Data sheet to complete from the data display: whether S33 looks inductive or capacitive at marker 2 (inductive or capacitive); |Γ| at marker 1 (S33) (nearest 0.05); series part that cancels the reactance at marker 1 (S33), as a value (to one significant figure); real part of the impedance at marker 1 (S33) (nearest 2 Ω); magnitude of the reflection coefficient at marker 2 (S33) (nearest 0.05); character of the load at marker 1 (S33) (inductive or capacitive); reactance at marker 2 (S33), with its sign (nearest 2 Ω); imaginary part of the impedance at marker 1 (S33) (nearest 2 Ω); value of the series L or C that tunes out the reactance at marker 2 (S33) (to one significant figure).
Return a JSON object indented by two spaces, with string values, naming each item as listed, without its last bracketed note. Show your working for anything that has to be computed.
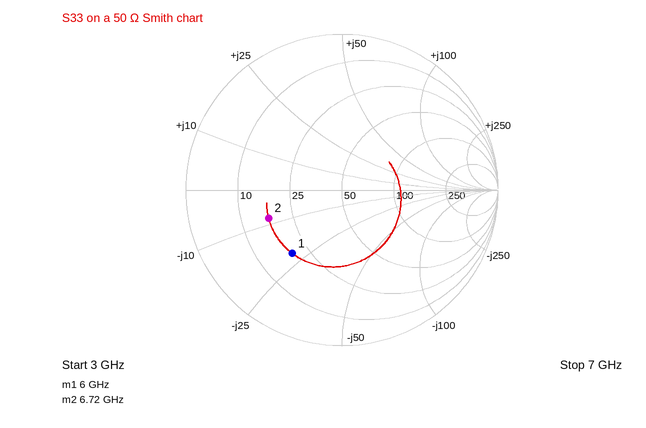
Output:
{
  "whether S33 looks inductive or capacitive at marker 2": "capacitive",
  "|Γ| at marker 1 (S33)": "0.50",
  "series part that cancels the reactance at marker 1 (S33), as a value": "L = 22 Ω/(2π × 6 GHz) ≈ 584 pH, so 600 pH to one significant figure",
  "real part of the impedance at marker 1 (S33)": "20 Ω",
  "magnitude of the reflection coefficient at marker 2 (S33)": "0.50",
  "character of the load at marker 1 (S33)": "capacitive",
  "reactance at marker 2 (S33), with its sign": "-8 Ω",
  "imaginary part of the impedance at marker 1 (S33)": "-22 Ω",
  "value of the series L or C that tunes out the reactance at marker 2 (S33)": "L = 8 Ω/(2π × 6.72 GHz) ≈ 189 pH, so 200 pH to one significant figure"
}
